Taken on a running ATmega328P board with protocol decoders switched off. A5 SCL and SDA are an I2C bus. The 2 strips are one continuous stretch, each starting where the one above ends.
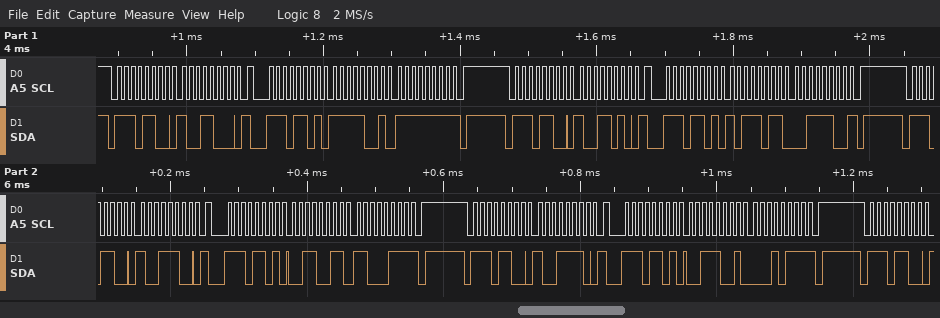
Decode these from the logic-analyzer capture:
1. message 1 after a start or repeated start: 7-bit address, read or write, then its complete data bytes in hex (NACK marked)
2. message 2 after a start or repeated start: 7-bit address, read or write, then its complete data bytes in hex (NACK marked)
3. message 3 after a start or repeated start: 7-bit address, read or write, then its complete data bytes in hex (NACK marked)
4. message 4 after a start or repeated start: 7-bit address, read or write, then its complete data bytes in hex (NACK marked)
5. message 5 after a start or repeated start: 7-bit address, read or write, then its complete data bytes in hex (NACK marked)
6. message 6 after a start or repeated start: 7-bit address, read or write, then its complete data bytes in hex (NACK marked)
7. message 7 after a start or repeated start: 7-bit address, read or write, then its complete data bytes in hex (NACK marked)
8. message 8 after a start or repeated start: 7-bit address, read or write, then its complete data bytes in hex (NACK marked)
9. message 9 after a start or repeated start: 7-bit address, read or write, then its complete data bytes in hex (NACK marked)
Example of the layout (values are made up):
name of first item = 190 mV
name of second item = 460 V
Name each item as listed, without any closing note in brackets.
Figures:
message 1 after a start or repeated start: 7-bit address, read or write, then its complete data bytes in hex = 0x76 write: 98
message 2 after a start or repeated start: 7-bit address, read or write, then its complete data bytes in hex = 0x76 read: F9 FF NACK
message 3 after a start or repeated start: 7-bit address, read or write, then its complete data bytes in hex = 0x76 write: 9A
message 4 after a start or repeated start: 7-bit address, read or write, then its complete data bytes in hex = 0x76 read: BB 3C NACK
message 5 after a start or repeated start: 7-bit address, read or write, then its complete data bytes in hex = 0x76 write: 9C
message 6 after a start or repeated start: 7-bit address, read or write, then its complete data bytes in hex = 0x76 read: 33 C7 NACK
message 7 after a start or repeated start: 7-bit address, read or write, then its complete data bytes in hex = 0x76 write: 9E
message 8 after a start or repeated start: 7-bit address, read or write, then its complete data bytes in hex = 0x76 read: 39 17 NACK
message 9 after a start or repeated start: 7-bit address, read or write, then its complete data bytes in hex = 0x76 write
